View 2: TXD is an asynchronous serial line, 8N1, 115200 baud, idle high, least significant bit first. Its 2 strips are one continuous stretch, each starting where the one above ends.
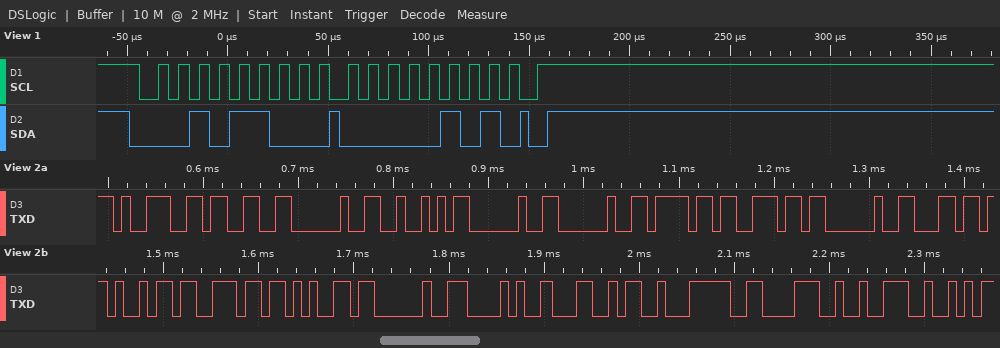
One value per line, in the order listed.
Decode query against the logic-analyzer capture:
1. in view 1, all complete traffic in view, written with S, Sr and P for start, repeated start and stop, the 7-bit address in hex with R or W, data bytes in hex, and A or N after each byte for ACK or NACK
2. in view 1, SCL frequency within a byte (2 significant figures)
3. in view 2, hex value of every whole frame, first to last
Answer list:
S 16W A 05 A P
100 kHz
0x39 0x33 0x20 0x52 0x20 0x20 0x6F 0x6E 0x20 0x6C 0x69 0x6E 0x65 0x20 0x28 0x4C 0xE2 0x86 0x92 0x52
